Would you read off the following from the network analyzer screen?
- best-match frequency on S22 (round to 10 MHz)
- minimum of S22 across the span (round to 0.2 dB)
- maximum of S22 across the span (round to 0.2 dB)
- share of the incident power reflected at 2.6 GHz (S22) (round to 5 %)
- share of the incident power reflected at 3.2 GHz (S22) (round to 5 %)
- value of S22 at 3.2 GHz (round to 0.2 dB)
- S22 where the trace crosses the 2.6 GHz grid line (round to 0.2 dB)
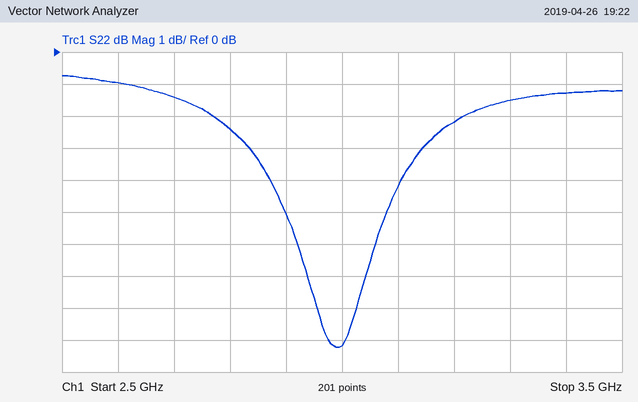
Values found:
2.99 GHz
-9.2 dB
-0.8 dB
80 %
60 %
-2.2 dB
-1.0 dB
